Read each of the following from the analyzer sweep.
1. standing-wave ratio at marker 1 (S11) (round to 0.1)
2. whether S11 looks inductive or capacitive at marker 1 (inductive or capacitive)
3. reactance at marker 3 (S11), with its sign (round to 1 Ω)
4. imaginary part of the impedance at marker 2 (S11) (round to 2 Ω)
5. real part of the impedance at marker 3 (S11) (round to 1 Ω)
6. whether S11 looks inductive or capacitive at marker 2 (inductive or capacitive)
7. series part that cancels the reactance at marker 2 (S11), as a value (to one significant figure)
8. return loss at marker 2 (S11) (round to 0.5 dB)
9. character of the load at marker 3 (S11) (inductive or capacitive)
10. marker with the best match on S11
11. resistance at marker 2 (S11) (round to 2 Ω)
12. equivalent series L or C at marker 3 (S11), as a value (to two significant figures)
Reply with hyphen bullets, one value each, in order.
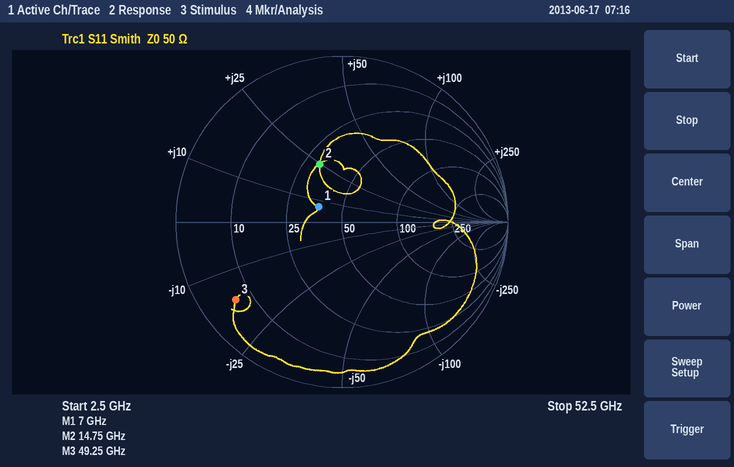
- 1.4
- inductive
- -16 Ω
- +24 Ω
- 6 Ω
- inductive
- 400 fF
- 8.5 dB
- capacitive
- marker 1
- 30 Ω
- 200 fF
